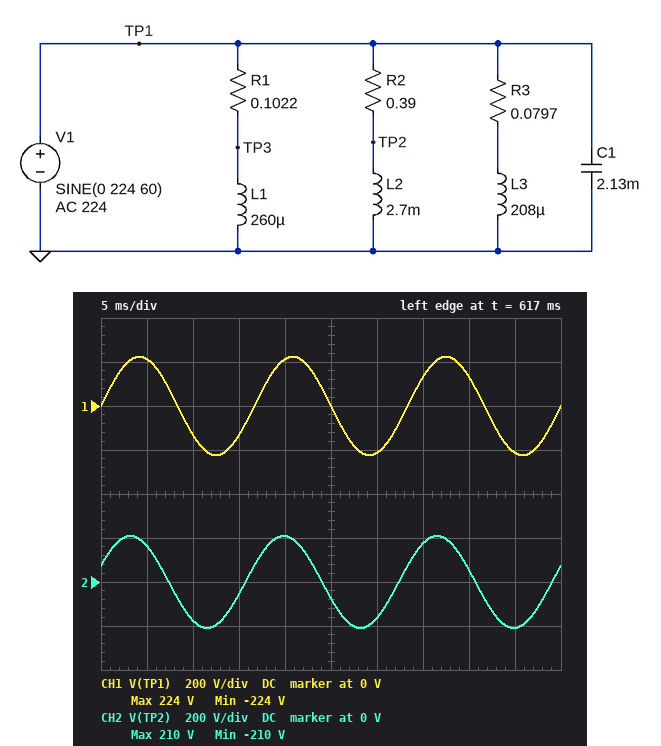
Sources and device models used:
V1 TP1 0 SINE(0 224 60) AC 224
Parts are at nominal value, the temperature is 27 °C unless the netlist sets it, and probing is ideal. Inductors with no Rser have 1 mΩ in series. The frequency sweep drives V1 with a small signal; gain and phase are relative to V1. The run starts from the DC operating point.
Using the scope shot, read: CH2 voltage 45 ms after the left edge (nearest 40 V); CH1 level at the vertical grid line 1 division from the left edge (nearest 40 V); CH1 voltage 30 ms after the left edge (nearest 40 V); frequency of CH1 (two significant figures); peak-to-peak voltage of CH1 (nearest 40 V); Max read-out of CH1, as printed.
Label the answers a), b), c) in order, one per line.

a) -200 V
b) 200 V
c) -200 V
d) 60 Hz
e) 440 V
f) 224 V
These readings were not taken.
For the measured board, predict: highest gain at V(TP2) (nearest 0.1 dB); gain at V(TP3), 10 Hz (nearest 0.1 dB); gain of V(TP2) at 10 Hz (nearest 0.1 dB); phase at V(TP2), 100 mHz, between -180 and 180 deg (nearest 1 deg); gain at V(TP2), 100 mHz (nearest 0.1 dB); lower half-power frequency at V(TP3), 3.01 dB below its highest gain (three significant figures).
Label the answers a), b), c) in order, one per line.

a) 0 dB
b) -16.1 dB
c) -8.0 dB
d) 59 deg
e) -46.0 dB
f) 63.2 Hz
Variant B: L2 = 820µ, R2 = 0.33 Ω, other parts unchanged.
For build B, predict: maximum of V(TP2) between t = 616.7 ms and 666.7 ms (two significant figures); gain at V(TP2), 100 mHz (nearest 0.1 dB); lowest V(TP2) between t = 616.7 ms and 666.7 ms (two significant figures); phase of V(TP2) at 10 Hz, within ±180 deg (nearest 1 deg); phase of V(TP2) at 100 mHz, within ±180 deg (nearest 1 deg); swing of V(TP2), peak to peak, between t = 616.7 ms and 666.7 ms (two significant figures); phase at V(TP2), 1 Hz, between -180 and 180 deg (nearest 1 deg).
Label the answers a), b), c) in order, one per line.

a) 150 V
b) -49.4 dB
c) -150 V
d) 80 deg
e) 27 deg
f) 310 V
g) 78 deg
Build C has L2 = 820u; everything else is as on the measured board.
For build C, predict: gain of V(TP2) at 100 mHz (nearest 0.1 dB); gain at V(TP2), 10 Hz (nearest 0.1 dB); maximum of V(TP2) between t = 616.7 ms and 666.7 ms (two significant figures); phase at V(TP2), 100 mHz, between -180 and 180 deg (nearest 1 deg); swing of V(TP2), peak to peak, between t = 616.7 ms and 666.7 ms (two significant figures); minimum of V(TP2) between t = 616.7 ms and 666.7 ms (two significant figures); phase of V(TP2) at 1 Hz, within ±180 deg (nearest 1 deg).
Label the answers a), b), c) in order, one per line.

a) -50.8 dB
b) -17.7 dB
c) 140 V
d) 27 deg
e) 280 V
f) -140 V
g) 78 deg
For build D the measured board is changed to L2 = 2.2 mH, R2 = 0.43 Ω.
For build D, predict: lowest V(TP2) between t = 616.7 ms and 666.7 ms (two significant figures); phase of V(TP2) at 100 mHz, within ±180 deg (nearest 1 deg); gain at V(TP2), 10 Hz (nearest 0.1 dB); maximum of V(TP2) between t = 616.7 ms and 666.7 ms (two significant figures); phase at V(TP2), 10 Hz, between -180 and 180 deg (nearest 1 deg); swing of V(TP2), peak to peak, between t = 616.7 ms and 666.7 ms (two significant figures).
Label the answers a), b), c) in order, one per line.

a) -200 V
b) 54 deg
c) -10.3 dB
d) 200 V
e) 72 deg
f) 400 V
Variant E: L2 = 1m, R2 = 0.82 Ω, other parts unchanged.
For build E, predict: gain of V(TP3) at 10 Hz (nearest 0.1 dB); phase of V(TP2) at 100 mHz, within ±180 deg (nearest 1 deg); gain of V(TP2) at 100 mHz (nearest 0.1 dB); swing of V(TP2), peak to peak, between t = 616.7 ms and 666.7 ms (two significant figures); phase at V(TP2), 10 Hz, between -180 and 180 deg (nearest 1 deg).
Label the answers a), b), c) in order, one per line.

a) -16.1 dB
b) 32 deg
c) -56.8 dB
d) 190 V
e) 85 deg
